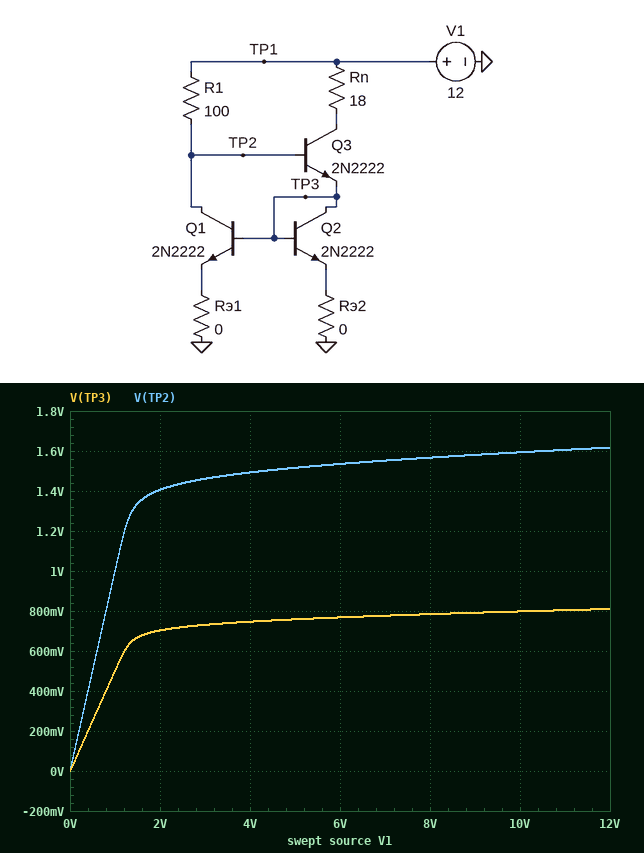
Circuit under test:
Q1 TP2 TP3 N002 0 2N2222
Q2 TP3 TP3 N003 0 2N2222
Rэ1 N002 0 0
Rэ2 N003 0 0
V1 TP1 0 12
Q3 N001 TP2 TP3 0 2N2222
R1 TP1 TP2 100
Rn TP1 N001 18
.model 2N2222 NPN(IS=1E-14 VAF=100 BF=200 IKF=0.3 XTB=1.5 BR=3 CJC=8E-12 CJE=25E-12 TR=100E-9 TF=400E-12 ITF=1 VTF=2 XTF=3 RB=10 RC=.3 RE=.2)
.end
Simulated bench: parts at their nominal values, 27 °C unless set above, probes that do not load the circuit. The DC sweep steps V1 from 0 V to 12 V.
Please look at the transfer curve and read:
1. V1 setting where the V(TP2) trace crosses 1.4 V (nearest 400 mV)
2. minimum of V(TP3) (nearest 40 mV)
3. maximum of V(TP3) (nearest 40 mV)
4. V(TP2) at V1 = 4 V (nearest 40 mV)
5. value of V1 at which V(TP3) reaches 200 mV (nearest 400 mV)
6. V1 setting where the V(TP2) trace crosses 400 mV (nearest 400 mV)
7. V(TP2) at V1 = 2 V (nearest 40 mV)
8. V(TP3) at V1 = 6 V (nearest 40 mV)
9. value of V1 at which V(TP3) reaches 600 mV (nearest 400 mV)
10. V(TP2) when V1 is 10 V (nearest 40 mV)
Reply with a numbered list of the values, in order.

1. 2.0 V
2. 0 V
3. 800 mV
4. 1.48 V
5. 400 mV
6. 400 mV
7. 1.40 V
8. 760 mV
9. 1.2 V
10. 1.60 V
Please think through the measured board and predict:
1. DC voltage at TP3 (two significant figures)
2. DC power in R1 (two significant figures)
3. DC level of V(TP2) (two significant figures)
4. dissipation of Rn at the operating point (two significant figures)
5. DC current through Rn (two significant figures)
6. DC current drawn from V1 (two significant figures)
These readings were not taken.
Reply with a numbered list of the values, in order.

1. 810 mV
2. 1.1 W
3. 1.6 V
4. 190 mW
5. 100 mA
6. 210 mA
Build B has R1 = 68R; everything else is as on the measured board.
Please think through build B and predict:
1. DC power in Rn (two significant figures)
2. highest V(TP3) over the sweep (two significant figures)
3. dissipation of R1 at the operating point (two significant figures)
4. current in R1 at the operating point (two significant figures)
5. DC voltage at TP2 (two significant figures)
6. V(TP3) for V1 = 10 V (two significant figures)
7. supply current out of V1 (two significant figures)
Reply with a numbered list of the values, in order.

1. 410 mW
2. 840 mV
3. 1.6 W
4. 150 mA
5. 1.7 V
6. 820 mV
7. 300 mA
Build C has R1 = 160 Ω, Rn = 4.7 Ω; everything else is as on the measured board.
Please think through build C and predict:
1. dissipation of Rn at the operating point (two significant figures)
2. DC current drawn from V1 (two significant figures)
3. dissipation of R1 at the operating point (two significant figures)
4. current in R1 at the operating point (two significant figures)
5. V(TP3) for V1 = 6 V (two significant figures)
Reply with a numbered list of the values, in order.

1. 20 mW
2. 130 mA
3. 680 mW
4. 65 mA
5. 750 mV
